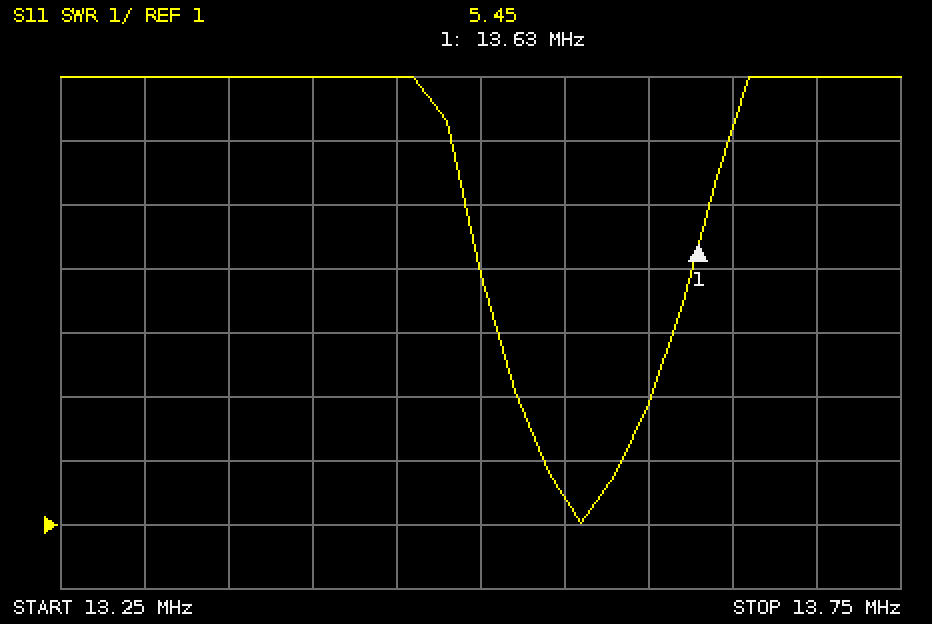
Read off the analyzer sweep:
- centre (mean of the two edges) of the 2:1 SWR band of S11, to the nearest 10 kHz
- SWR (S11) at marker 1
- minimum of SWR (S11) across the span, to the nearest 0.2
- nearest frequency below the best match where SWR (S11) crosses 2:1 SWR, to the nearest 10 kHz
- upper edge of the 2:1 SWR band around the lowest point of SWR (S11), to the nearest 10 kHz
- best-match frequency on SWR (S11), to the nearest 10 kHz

13.56 MHz
5.45
1.0
13.54 MHz
13.58 MHz
13.56 MHz
